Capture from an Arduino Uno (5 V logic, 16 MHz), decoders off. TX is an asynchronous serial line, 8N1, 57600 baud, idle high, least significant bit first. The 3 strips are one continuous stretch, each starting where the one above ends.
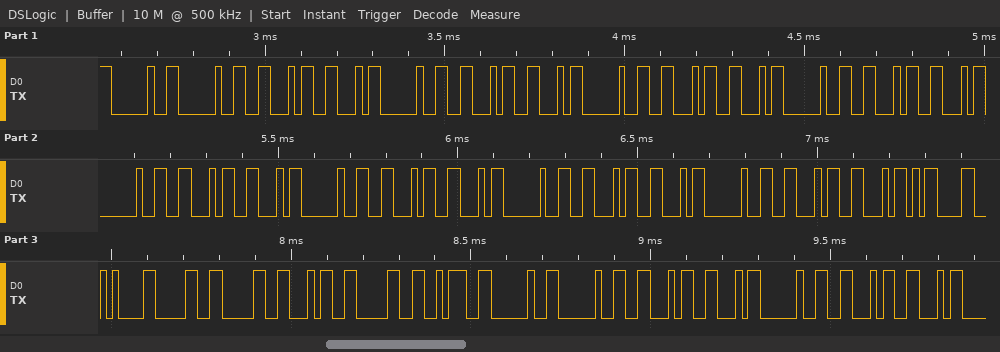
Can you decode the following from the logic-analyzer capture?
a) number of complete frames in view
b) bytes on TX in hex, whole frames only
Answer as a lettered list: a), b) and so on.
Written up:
a) 39
b) 0x20 0x20 0x46 0x46 0x20 0x46 0x46 0x20 0x46 0x46 0x20 0x46 0x46 0x20 0x46 0x46 0x20 0x46 0x46 0x20 0x46 0x46 0x20 0x46 0x46 0x0D 0x0A 0x30 0x30 0x34 0x30 0x3A 0x20 0x20 0x46 0x46 0x20 0x46 0x46
